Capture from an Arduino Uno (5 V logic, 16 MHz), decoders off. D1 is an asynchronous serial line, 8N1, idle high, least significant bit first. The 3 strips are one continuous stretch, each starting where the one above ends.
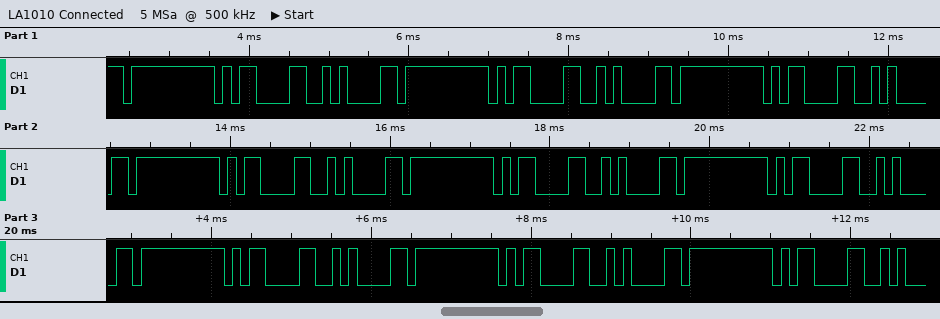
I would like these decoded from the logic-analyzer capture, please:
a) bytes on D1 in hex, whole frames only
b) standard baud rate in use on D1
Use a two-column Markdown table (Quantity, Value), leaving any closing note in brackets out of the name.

| Quantity | Value |
|---|---|
| bytes on D1 in hex, whole frames only | 0xFF 0x0D 0x0A 0xFF 0x0D 0x0A 0xFF 0x0D 0x0A 0xFF 0x0D 0x0A 0xFF 0x0D 0x0A 0xFF 0x0D 0x0A 0xFF 0x0D 0x0A 0xFF 0x0D 0x0A 0xFF 0x0D |
| standard baud rate in use on D1 | 9600 baud |
